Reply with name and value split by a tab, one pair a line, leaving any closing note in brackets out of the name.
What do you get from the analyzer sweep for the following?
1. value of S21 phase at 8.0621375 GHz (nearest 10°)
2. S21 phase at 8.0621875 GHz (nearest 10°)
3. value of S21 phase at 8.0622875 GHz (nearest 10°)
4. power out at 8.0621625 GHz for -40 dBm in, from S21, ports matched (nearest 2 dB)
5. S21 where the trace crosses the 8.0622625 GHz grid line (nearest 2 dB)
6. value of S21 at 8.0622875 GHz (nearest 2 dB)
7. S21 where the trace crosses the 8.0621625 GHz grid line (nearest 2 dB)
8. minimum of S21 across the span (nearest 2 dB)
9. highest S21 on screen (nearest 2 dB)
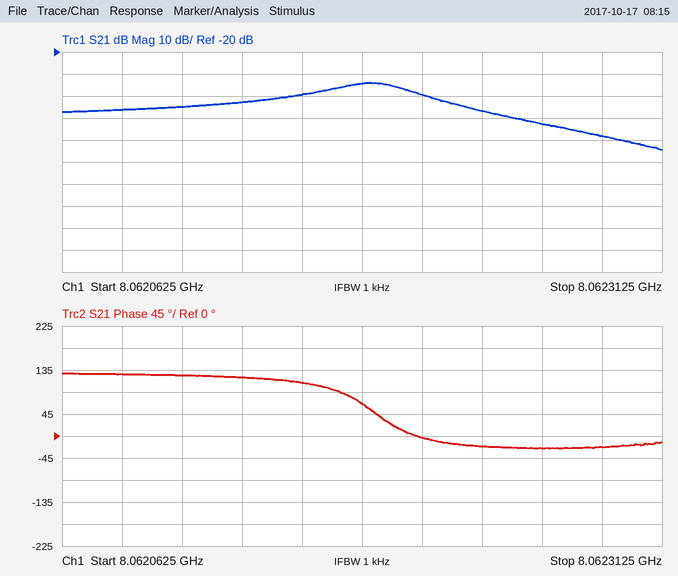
value of S21 phase at 8.0621375 GHz	120°
S21 phase at 8.0621875 GHz	70°
value of S21 phase at 8.0622875 GHz	-20°
power out at 8.0621625 GHz for -40 dBm in, from S21, ports matched	-80 dBm
S21 where the trace crosses the 8.0622625 GHz grid line	-52 dB
value of S21 at 8.0622875 GHz	-58 dB
S21 where the trace crosses the 8.0621625 GHz grid line	-40 dB
minimum of S21 across the span	-64 dB
highest S21 on screen	-34 dB
